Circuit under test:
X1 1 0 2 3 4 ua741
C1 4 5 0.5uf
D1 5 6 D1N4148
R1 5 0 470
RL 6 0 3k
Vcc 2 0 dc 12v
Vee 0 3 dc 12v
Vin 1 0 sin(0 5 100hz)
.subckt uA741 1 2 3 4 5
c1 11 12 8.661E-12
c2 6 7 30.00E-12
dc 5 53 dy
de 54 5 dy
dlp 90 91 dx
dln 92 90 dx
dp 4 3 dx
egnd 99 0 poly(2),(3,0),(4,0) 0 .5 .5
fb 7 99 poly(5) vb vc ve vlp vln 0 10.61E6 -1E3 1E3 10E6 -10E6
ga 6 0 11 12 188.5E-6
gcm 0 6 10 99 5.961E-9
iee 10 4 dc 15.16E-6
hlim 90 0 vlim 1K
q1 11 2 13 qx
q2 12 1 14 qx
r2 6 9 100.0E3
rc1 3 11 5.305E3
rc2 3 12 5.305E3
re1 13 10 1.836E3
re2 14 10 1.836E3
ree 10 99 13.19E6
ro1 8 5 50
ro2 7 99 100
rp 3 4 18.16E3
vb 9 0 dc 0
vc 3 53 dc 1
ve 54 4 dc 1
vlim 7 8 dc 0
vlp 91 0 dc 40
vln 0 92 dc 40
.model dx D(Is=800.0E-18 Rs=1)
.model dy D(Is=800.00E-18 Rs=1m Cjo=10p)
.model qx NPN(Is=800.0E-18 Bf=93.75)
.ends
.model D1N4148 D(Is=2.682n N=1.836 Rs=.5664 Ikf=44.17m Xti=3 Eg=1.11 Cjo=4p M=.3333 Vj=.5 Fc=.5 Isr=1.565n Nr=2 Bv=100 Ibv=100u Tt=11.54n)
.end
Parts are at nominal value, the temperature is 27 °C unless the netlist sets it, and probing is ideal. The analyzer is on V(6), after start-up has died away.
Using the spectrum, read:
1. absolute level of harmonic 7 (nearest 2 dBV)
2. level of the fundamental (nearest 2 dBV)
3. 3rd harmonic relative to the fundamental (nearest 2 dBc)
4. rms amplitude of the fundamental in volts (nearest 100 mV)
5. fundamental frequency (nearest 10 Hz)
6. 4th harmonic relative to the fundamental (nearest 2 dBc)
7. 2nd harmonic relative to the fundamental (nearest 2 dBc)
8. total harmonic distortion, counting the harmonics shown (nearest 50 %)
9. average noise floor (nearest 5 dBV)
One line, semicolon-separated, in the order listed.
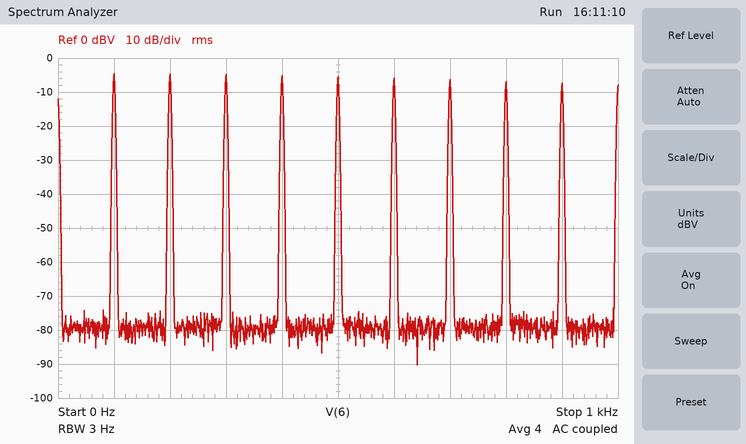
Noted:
-6 dBV; -4 dBV; 0 dBc; 600 mV; 100 Hz; 0 dBc; 0 dBc; 250 %; -80 dBV
